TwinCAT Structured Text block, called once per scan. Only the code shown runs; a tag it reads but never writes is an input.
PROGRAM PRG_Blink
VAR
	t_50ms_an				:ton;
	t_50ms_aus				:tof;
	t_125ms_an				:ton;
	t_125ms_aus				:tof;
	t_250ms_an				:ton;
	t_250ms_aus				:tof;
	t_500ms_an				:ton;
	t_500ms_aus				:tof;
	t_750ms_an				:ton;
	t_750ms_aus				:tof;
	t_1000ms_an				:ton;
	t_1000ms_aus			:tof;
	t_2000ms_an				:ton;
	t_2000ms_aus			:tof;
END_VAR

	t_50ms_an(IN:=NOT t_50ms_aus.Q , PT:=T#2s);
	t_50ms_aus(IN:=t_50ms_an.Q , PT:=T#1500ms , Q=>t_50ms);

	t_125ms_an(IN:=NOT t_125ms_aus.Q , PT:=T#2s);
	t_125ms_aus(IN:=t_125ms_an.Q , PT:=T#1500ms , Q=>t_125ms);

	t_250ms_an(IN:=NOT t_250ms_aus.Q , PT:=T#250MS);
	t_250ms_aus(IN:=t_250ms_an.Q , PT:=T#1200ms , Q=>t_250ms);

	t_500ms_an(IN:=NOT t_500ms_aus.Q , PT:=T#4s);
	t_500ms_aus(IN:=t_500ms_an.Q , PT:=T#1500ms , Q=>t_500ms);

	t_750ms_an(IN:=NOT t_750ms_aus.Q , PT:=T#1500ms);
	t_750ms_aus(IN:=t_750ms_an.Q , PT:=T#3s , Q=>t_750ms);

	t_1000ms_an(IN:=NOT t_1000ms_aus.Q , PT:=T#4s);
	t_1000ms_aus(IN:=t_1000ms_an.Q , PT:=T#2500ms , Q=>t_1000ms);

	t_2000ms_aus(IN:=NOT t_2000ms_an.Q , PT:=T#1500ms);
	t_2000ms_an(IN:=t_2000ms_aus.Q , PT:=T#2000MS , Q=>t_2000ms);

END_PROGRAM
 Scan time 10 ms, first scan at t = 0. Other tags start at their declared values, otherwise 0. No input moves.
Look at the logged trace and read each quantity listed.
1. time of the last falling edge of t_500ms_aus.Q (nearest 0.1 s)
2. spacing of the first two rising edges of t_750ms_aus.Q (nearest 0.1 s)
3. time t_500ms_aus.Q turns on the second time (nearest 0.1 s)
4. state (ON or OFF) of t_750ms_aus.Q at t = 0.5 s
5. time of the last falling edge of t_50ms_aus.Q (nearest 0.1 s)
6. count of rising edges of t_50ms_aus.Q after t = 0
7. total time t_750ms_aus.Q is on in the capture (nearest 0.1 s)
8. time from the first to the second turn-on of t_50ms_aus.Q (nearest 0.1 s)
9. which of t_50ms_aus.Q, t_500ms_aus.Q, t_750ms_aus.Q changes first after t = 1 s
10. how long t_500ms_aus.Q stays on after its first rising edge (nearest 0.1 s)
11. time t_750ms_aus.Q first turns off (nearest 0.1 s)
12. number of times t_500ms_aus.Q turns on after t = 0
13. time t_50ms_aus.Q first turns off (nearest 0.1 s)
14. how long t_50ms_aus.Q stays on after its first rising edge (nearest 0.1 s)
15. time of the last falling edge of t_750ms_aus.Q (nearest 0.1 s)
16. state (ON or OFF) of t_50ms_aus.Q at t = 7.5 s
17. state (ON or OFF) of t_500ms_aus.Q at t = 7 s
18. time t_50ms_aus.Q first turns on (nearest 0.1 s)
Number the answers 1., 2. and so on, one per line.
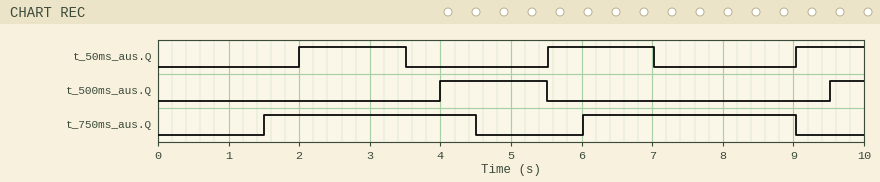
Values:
1. 5.5 s
2. 4.5 s
3. 9.5 s
4. OFF
5. 7.0 s
6. 3
7. 6.0 s
8. 3.5 s
9. t_750ms_aus.Q
10. 1.5 s
11. 4.5 s
12. 2
13. 3.5 s
14. 1.5 s
15. 9.0 s
16. OFF
17. OFF
18. 2.0 s
